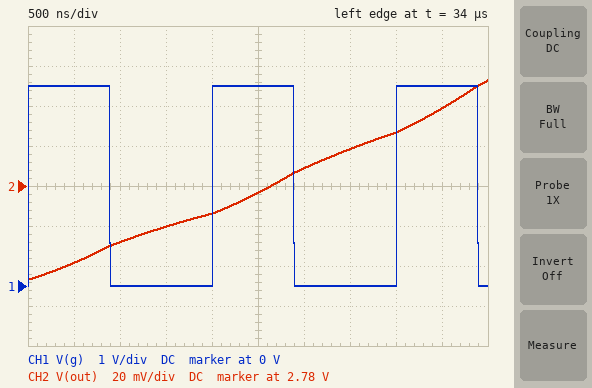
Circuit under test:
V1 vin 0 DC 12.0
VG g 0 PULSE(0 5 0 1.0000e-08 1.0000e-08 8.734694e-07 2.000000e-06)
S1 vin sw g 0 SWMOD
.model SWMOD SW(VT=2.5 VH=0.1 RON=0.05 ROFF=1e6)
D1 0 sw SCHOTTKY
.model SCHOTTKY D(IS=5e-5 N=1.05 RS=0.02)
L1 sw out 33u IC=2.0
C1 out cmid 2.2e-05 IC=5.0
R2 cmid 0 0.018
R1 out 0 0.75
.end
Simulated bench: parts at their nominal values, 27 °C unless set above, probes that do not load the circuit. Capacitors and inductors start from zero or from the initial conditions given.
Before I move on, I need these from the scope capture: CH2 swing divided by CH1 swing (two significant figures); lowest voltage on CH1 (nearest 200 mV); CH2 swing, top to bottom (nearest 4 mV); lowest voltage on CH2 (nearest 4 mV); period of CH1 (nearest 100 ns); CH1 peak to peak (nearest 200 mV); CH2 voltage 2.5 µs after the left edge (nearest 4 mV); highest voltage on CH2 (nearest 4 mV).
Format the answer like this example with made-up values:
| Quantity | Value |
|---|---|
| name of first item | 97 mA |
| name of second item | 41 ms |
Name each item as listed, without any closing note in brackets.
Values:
| Quantity | Value |
|---|---|
| CH2 swing divided by CH1 swing | 0.020 |
| lowest voltage on CH1 | 0 V |
| CH2 swing, top to bottom | 100 mV |
| lowest voltage on CH2 | 2.732 V |
| period of CH1 | 2.0 µs |
| CH1 peak to peak | 5.0 V |
| CH2 voltage 2.5 µs after the left edge | 2.776 V |
| highest voltage on CH2 | 2.832 V |
